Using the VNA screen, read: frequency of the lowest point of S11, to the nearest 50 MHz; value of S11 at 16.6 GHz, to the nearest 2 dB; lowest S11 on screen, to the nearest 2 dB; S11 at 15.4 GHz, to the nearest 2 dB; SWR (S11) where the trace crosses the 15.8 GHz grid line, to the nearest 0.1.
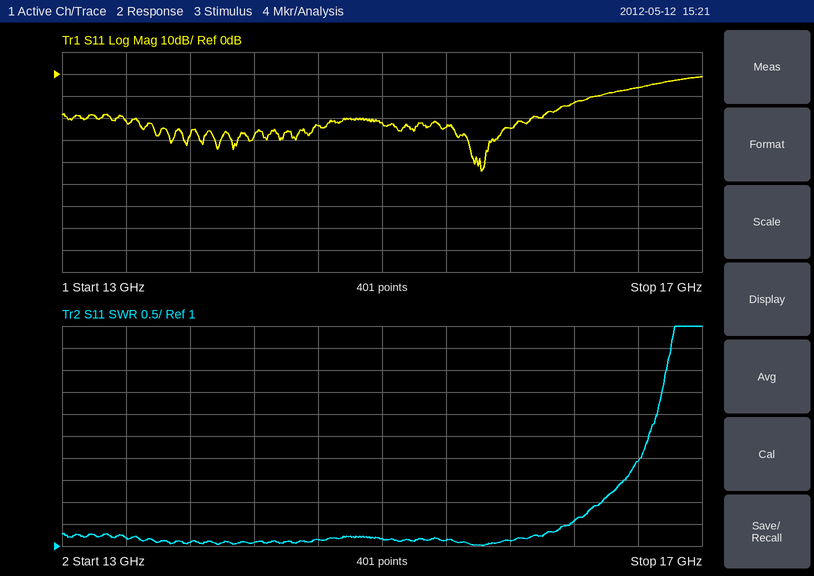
15.60 GHz
-6 dB
-44 dB
-24 dB
1.1
